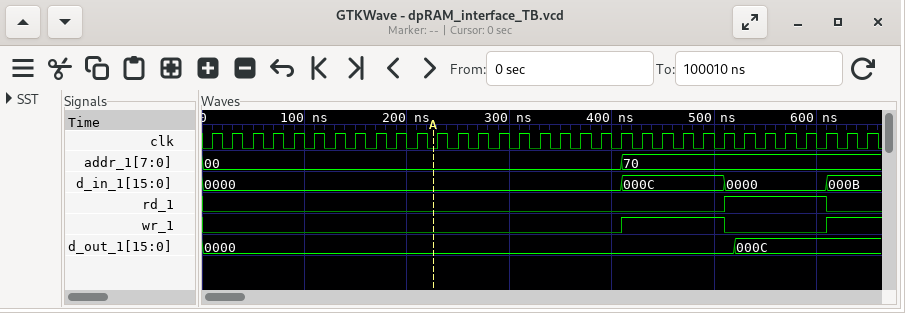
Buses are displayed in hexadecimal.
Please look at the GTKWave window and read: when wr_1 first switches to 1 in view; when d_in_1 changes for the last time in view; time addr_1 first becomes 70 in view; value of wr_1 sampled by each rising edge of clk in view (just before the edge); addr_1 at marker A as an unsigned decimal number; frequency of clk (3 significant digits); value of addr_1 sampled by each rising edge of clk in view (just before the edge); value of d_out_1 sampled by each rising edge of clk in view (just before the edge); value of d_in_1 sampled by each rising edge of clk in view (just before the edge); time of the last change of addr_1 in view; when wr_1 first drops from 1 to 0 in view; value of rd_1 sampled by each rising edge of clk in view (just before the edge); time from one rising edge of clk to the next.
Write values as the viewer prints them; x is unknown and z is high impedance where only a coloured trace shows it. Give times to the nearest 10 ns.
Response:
410 ns
610 ns
410 ns
0 0 0 0 0 0 0 0 0 0 0 0 0 0 0 0 0 0 0 0 0 1 1 1 1 1 0 0 0 0 0 1 1
0
50.0 MHz
00, 00, 00, 00, 00, 00, 00, 00, 00, 00, 00, 00, 00, 00, 00, 00, 00, 00, 00, 00, 00, 70, 70, 70, 70, 70, 70, 70, 70, 70, 70, 70, 70
0000, 0000, 0000, 0000, 0000, 0000, 0000, 0000, 0000, 0000, 0000, 0000, 0000, 0000, 0000, 0000, 0000, 0000, 0000, 0000, 0000, 0000, 0000, 0000, 0000, 0000, 000C, 000C, 000C, 000C, 000C, 000C, 000C
0000, 0000, 0000, 0000, 0000, 0000, 0000, 0000, 0000, 0000, 0000, 0000, 0000, 0000, 0000, 0000, 0000, 0000, 0000, 0000, 0000, 000C, 000C, 000C, 000C, 000C, 0000, 0000, 0000, 0000, 0000, 000B, 000B
410 ns
510 ns
0 0 0 0 0 0 0 0 0 0 0 0 0 0 0 0 0 0 0 0 0 0 0 0 0 0 1 1 1 1 1 0 0
20 ns
